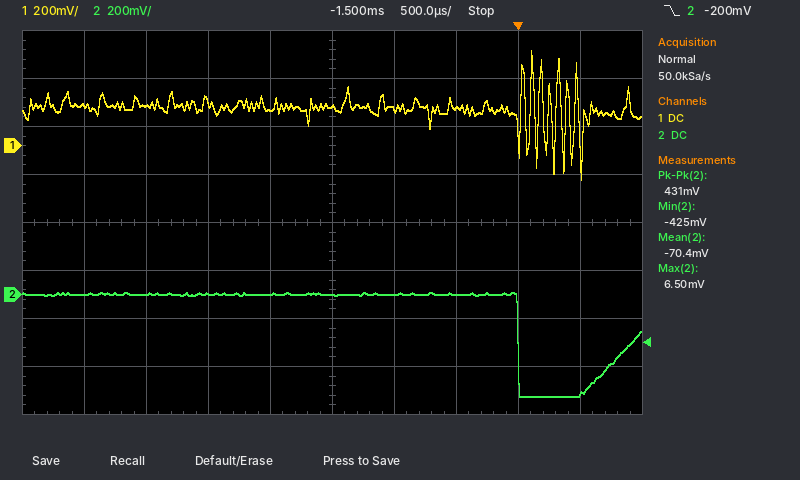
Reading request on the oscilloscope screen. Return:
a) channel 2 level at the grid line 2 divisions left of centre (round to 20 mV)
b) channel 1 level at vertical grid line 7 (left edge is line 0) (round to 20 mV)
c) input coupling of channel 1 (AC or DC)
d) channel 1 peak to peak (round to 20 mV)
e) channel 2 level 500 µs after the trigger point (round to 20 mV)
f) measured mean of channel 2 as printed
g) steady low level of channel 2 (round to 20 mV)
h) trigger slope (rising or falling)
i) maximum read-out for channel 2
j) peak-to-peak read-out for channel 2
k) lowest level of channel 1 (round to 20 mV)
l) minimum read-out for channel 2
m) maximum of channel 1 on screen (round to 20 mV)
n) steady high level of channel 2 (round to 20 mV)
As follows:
0 mV
160 mV
DC
540 mV
-420 mV
-70.4 mV
-420 mV
falling
6.50 mV
431 mV
-140 mV
-425 mV
400 mV
0 mV
